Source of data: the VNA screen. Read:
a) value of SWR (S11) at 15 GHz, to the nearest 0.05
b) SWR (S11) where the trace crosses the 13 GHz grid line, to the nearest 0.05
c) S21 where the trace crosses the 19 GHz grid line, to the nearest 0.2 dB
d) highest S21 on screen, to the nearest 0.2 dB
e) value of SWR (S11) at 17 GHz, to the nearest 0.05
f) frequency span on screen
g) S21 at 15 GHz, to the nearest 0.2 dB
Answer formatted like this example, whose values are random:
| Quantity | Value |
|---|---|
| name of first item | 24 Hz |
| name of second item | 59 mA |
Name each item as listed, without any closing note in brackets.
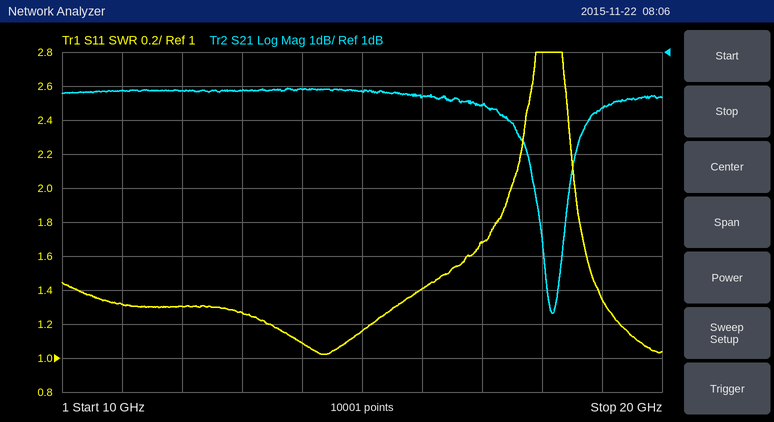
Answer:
| Quantity | Value |
|---|---|
| value of SWR (S11) at 15 GHz, to the nearest 0.05 | 1.15 |
| SWR (S11) where the trace crosses the 13 GHz grid line, to the nearest 0.05 | 1.25 |
| S21 where the trace crosses the 19 GHz grid line, to the nearest 0.2 dB | -0.6 dB |
| highest S21 on screen, to the nearest 0.2 dB | 0.0 dB |
| value of SWR (S11) at 17 GHz, to the nearest 0.05 | 1.70 |
| frequency span on screen | 10 GHz |
| S21 at 15 GHz, to the nearest 0.2 dB | -0.2 dB |
